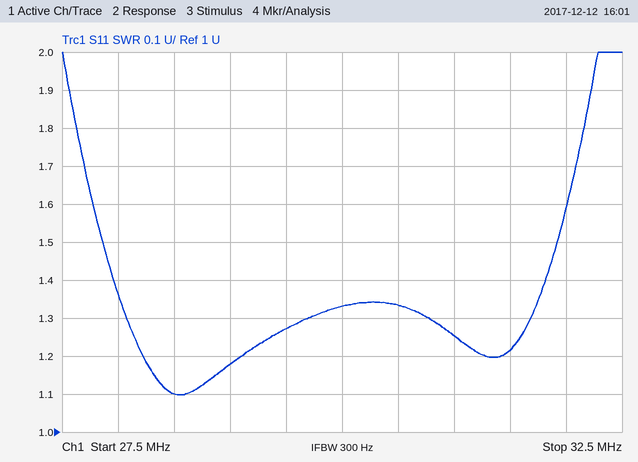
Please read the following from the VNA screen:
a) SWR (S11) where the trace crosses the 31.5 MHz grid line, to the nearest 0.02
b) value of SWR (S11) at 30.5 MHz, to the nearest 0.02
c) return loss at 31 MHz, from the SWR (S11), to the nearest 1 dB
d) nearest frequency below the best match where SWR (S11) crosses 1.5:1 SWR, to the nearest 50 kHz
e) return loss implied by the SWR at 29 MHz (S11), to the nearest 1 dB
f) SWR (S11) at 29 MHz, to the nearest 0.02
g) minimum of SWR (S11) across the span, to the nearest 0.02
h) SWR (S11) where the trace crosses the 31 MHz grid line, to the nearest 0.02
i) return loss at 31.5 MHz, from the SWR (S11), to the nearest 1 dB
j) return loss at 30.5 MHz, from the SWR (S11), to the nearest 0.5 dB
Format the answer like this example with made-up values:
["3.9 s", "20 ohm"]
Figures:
["1.22", "1.34", "19 dB", "27.85 MHz", "22 dB", "1.18", "1.10", "1.26", "20 dB", "17.0 dB"]
